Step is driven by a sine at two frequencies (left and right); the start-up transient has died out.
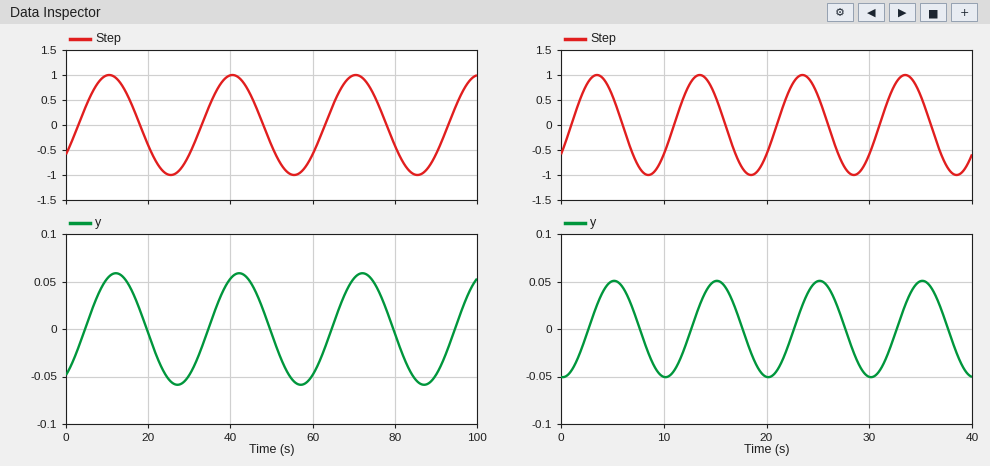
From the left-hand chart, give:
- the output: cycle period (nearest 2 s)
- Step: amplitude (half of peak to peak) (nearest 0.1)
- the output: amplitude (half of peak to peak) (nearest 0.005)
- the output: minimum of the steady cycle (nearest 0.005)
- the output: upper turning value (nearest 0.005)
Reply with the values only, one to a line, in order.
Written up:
30 s
1.0
0.060
-0.060
0.060
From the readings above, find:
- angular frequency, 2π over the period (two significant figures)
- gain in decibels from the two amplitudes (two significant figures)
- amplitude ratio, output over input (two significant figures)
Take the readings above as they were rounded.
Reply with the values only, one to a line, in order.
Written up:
0.21 rad/s
-24 dB
0.060
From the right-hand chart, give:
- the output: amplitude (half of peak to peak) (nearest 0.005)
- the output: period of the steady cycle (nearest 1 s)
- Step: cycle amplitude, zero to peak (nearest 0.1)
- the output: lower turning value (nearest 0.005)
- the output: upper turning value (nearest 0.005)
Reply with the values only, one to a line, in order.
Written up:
0.050
10 s
1.0
-0.050
0.050
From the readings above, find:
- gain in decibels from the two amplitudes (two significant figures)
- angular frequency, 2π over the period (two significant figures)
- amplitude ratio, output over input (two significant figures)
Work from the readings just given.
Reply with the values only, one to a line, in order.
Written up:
-26 dB
0.63 rad/s
0.050
